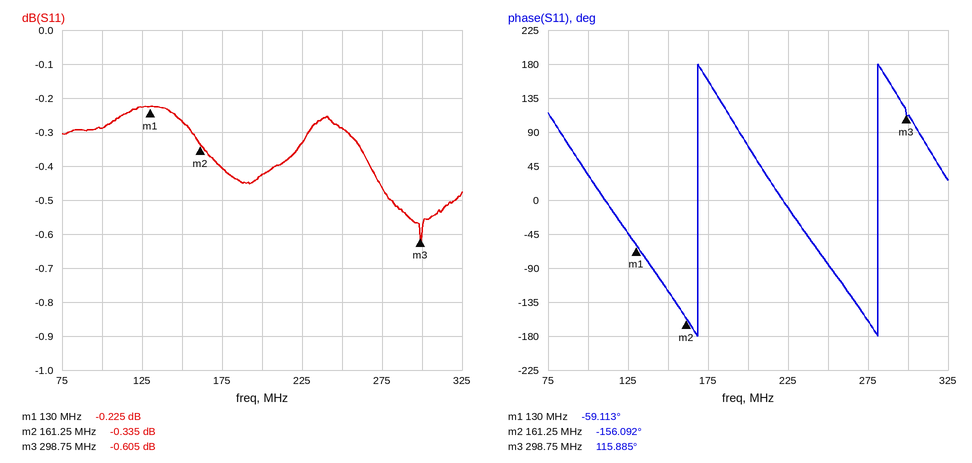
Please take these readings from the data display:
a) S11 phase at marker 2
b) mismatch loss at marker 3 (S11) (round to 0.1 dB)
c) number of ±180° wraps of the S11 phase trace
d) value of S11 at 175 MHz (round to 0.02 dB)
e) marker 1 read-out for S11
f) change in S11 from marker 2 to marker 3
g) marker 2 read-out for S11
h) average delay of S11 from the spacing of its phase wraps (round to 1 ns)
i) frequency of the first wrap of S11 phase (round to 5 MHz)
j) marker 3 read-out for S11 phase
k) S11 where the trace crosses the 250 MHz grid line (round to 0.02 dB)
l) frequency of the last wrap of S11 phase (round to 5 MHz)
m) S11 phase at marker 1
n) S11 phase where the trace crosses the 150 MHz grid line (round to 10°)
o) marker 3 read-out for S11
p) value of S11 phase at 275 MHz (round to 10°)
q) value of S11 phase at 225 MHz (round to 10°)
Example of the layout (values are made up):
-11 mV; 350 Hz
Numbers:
-156.092°; 8.9 dB; 2; -0.40 dB; -0.225 dB; -0.270 dB; -0.335 dB; 9 ns; 170 MHz; 115.885°; -0.28 dB; 280 MHz; -59.113°; -120°; -0.605 dB; -160°; -10°
